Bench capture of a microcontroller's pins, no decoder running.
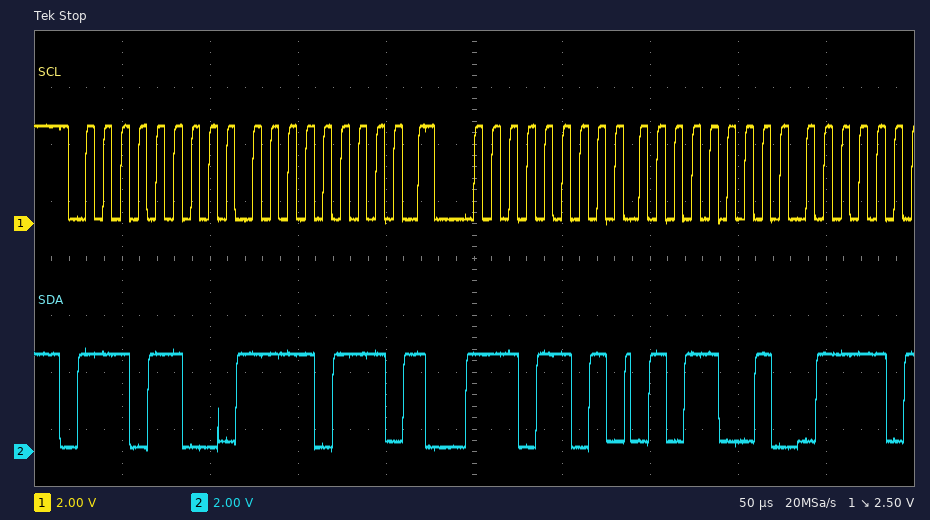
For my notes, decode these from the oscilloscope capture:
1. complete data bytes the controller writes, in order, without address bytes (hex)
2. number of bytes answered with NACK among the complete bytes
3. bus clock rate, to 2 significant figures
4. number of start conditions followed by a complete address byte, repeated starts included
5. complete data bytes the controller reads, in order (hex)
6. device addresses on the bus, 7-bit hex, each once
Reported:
F7
0
100 kHz
2
59
0x76
